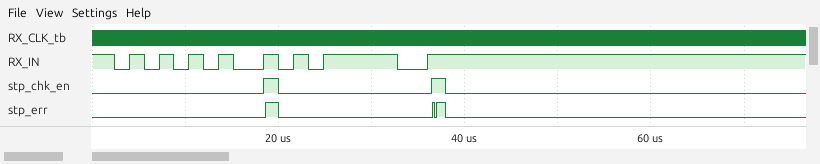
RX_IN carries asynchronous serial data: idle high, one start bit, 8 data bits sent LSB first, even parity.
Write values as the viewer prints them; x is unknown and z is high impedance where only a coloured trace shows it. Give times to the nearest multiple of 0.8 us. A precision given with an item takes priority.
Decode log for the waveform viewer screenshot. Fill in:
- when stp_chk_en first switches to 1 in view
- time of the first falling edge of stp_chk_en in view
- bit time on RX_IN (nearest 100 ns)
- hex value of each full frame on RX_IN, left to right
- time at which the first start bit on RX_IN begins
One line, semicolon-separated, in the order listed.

18.4 us; 20 us; 1600 ns; 55, 7D; 2.4 us
